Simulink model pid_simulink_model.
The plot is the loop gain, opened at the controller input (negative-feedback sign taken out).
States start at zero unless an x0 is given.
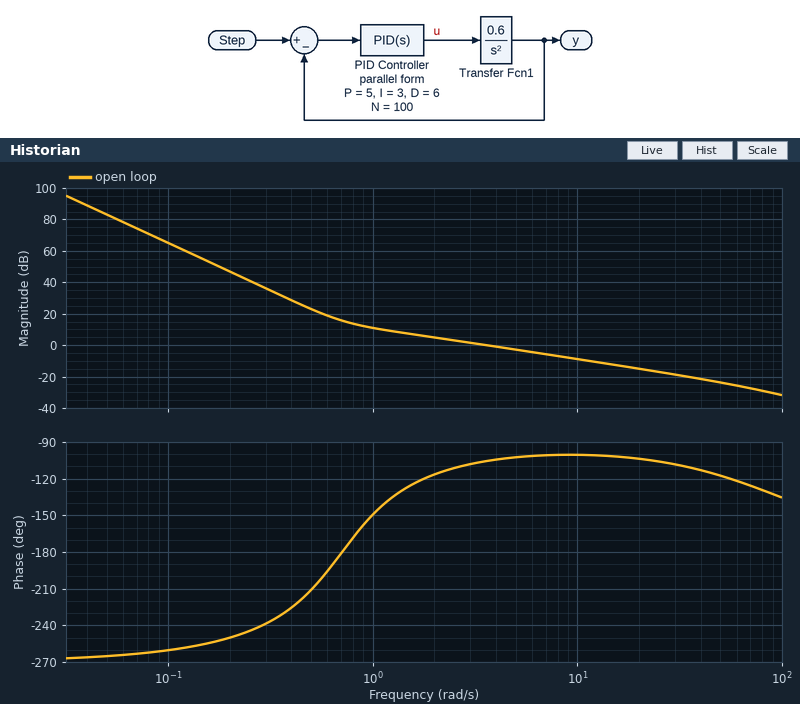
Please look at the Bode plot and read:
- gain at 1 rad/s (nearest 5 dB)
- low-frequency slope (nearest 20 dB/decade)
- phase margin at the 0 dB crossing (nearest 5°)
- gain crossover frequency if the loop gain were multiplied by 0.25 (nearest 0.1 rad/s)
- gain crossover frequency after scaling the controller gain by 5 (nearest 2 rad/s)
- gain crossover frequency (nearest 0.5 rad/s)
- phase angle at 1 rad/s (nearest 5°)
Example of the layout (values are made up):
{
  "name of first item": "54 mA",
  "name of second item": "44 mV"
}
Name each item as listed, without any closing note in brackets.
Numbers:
{
  "gain at 1 rad/s": "10 dB",
  "low-frequency slope": "-60 dB/decade",
  "phase margin at the 0 dB crossing": "75°",
  "gain crossover frequency if the loop gain were multiplied by 0.25": "0.9 rad/s",
  "gain crossover frequency after scaling the controller gain by 5": "18 rad/s",
  "gain crossover frequency": "3.5 rad/s",
  "phase angle at 1 rad/s": "-150°"
}
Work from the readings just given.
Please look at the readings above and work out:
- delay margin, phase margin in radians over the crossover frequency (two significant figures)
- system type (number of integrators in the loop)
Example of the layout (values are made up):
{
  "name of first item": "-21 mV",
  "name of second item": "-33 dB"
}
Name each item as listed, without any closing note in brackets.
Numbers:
{
  "delay margin, phase margin in radians over the crossover frequency": "0.37 s",
  "system type": "3"
}
